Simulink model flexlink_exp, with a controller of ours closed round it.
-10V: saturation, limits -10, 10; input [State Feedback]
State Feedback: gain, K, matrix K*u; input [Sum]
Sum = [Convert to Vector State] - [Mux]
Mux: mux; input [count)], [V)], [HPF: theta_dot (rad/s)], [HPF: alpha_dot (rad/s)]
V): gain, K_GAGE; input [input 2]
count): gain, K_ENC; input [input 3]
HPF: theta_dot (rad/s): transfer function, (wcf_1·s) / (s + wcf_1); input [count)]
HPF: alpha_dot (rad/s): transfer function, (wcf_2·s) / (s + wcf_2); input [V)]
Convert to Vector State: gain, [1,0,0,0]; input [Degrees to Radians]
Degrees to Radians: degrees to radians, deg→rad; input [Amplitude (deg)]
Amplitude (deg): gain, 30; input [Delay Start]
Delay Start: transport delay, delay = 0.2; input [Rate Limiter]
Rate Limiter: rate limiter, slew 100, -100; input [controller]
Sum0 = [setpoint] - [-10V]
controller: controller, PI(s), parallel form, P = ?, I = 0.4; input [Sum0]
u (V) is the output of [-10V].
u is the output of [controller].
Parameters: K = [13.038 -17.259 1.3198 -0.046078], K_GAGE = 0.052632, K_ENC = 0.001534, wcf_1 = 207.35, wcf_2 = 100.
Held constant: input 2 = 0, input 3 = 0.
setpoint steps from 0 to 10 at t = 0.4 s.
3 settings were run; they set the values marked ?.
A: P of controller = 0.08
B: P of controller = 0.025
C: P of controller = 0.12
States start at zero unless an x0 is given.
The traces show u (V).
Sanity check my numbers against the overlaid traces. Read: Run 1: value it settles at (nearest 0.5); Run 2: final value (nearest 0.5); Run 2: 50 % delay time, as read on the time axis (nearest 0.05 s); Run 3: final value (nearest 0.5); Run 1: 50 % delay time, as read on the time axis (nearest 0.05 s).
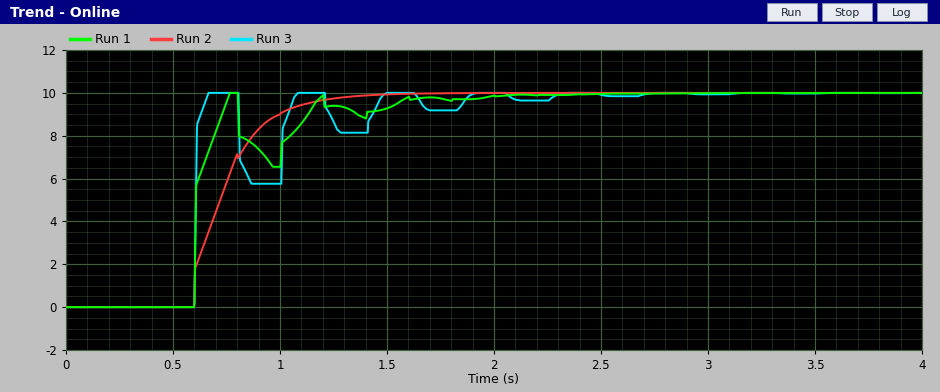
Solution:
10.0
10.0
0.70 s
10.0
0.60 s
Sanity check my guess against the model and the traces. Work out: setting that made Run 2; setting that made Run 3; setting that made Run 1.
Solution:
B
C
A
